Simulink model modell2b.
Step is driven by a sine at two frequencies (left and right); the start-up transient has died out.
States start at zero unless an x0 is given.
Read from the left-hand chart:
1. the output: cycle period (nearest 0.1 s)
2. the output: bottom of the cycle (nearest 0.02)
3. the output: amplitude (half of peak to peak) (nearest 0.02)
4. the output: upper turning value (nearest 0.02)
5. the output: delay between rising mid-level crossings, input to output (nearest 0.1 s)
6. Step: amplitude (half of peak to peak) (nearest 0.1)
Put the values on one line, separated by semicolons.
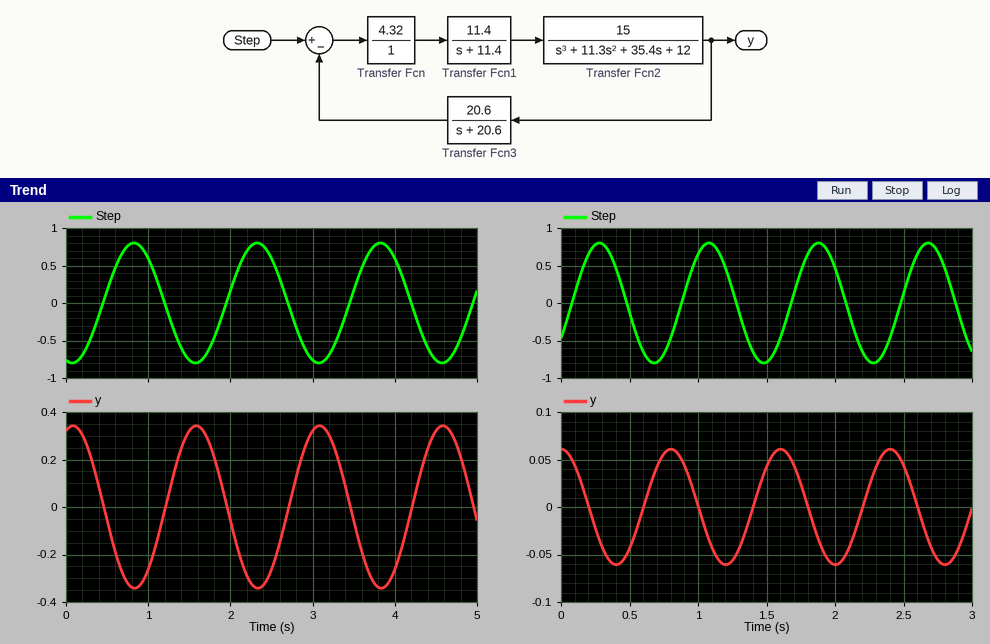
1.5 s; -0.34; 0.34; 0.34; 0.8 s; 0.8
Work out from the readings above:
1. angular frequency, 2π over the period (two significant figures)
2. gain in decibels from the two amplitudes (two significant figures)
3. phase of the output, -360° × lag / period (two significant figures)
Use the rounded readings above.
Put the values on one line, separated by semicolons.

4.2 rad/s; -7.4 dB; -190°
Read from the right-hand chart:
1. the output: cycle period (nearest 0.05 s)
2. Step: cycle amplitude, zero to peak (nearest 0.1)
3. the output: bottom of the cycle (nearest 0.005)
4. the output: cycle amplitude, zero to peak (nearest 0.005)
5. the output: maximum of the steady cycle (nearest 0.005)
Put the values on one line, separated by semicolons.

0.80 s; 0.8; -0.060; 0.060; 0.060
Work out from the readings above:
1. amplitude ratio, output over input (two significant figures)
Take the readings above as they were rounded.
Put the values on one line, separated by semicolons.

0.075
